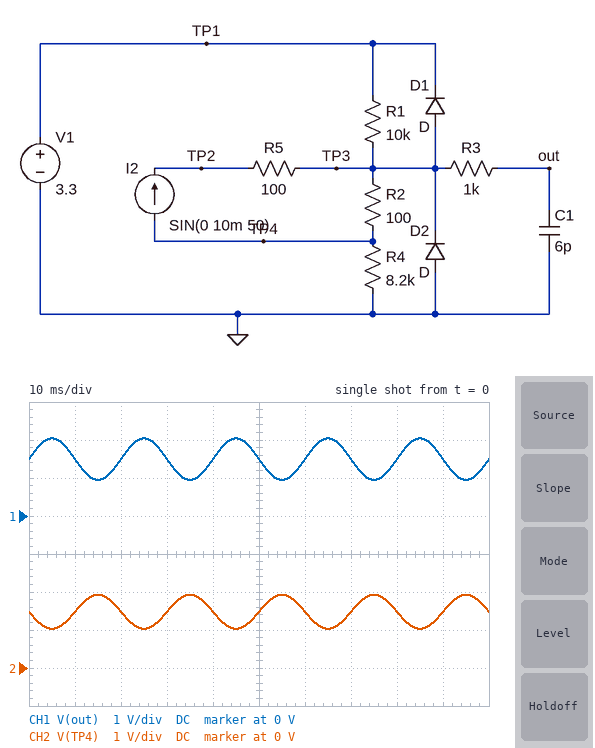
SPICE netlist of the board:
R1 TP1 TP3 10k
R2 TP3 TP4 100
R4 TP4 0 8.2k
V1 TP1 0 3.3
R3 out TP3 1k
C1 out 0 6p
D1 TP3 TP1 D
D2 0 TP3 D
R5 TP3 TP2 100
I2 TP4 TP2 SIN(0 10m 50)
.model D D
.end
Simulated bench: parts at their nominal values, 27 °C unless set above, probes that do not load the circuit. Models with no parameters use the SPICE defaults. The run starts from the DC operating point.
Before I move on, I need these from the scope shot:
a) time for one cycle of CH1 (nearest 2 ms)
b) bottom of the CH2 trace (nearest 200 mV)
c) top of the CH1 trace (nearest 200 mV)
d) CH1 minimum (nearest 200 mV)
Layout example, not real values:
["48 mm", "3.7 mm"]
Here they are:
["20 ms", "1.0 V", "2.0 V", "1.0 V"]
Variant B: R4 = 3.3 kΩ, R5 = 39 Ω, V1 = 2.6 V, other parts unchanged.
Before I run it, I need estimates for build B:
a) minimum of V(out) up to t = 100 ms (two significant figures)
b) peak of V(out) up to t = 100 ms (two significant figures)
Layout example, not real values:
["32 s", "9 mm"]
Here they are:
["-87 mV", "1.4 V"]
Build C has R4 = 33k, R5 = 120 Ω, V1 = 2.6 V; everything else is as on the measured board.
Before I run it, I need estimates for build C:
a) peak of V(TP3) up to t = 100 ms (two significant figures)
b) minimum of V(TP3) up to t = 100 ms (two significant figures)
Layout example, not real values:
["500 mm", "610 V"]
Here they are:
["2.2 V", "1.8 V"]
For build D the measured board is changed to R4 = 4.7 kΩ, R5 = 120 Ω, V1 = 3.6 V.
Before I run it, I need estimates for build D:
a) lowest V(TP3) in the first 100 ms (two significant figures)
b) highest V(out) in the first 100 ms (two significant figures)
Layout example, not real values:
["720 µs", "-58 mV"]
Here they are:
["490 mV", "1.8 V"]
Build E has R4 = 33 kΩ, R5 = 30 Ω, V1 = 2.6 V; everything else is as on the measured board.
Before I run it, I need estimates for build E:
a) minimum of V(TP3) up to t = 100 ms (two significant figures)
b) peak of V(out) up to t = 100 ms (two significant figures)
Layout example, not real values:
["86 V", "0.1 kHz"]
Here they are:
["1.8 V", "2.2 V"]
